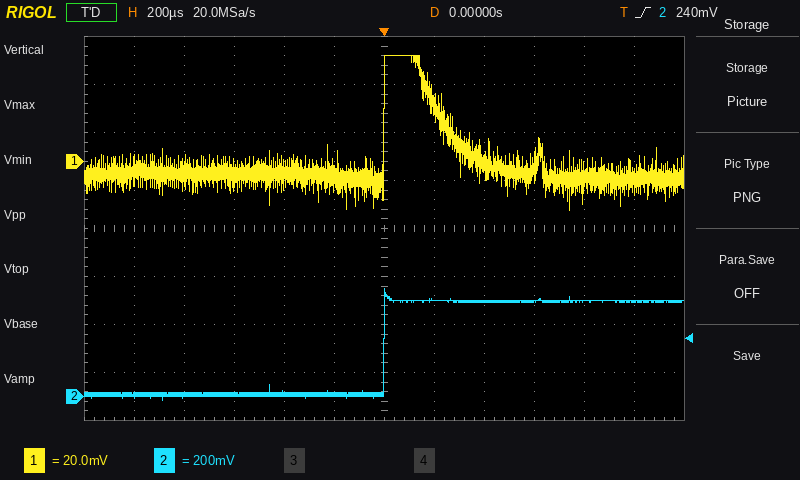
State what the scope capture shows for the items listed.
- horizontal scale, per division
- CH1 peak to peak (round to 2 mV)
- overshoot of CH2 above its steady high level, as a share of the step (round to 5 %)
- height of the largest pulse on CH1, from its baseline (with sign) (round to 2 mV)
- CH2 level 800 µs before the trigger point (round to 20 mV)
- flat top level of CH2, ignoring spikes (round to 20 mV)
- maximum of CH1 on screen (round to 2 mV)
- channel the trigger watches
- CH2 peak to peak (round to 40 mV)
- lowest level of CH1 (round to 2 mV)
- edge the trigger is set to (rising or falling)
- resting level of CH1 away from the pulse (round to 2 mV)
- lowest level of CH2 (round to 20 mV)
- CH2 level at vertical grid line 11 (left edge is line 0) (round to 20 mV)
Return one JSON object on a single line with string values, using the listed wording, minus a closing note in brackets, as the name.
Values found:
{"horizontal scale, per division": "200 µs", "CH1 peak to peak": "64 mV", "overshoot of CH2 above its steady high level, as a share of the step": "15 %", "height of the largest pulse on CH1, from its baseline (with sign)": "+50 mV", "CH2 level 800 µs before the trigger point": "0 mV", "flat top level of CH2, ignoring spikes": "400 mV", "maximum of CH1 on screen": "44 mV", "channel the trigger watches": "CH2", "CH2 peak to peak": "480 mV", "lowest level of CH1": "-20 mV", "edge the trigger is set to": "rising", "resting level of CH1 away from the pulse": "-6 mV", "lowest level of CH2": "-20 mV", "CH2 level at vertical grid line 11 (left edge is line 0)": "400 mV"}
